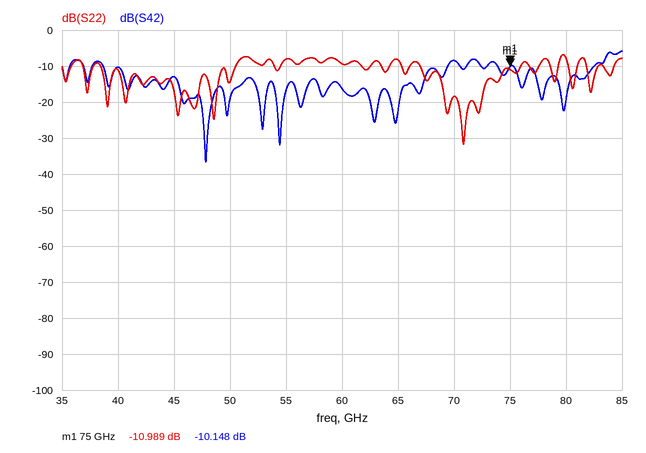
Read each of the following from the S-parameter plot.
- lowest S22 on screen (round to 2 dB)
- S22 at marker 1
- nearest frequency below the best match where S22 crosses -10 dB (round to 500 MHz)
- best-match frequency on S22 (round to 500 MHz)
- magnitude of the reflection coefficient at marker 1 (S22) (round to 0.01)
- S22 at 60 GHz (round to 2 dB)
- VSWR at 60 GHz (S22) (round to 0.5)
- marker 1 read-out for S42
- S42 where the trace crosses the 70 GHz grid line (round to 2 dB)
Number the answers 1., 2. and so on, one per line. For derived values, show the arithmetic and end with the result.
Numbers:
1. -32 dB
2. -10.989 dB
3. 67.0 GHz
4. 71.0 GHz
5. 10^(-10.989/20) ≈ 0.28
6. -10 dB
7. |Γ| = 10^(-10/20) = 0.3162; VSWR = (1 + 0.3162)/(1 − 0.3162) ≈ 1.92, so 2.0 to the nearest 0.5
8. -10.148 dB
9. -8 dB
